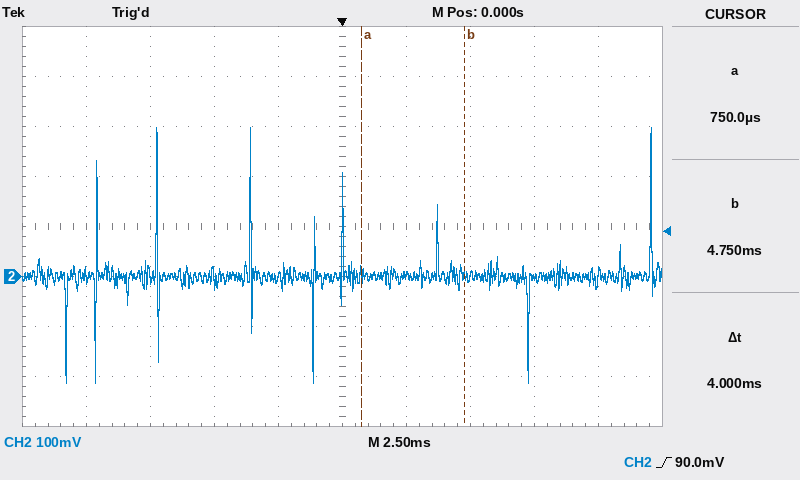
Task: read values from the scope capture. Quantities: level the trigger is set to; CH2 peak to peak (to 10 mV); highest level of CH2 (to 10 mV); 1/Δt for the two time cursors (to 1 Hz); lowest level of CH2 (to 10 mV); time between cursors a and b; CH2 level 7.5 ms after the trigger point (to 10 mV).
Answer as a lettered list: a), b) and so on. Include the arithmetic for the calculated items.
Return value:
a) 90.0 mV
b) 300 mV − (-210 mV) = 510 mV
c) 300 mV
d) 1 / 4 ms ≈ 250 Hz
e) -210 mV
f) 4 ms
g) 0 mV
